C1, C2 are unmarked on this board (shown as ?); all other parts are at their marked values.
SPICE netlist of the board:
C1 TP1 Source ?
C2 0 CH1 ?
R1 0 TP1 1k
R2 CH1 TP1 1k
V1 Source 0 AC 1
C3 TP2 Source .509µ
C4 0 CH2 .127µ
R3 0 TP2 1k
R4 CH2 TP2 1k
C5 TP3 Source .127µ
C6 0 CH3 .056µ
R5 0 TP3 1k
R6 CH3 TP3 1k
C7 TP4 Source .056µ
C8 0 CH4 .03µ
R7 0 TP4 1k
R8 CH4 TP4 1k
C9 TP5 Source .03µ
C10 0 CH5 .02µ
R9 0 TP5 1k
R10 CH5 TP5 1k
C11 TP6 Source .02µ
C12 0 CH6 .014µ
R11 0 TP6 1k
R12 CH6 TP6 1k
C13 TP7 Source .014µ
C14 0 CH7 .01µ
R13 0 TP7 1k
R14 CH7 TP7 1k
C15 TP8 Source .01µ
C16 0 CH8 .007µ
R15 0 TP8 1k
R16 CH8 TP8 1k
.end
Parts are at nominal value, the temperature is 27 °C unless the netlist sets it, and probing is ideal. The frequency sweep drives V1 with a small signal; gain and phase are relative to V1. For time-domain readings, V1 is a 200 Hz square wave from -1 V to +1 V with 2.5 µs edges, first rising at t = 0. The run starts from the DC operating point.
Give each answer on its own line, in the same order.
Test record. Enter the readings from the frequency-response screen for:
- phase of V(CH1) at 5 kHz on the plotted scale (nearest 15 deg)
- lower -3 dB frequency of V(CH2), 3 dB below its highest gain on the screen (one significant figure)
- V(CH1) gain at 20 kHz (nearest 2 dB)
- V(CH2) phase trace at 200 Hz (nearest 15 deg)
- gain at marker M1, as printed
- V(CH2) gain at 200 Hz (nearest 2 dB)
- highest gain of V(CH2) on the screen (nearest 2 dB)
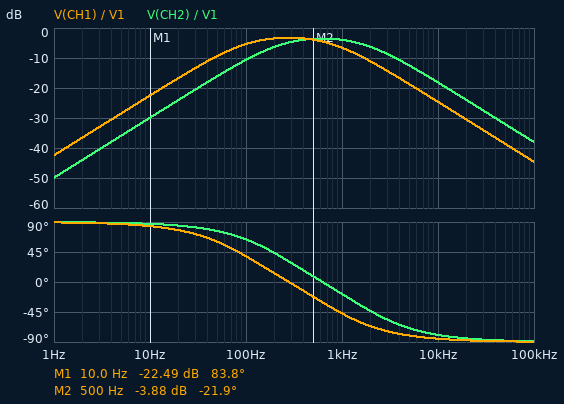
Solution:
-75 deg
200 Hz
-30 dB
45 deg
-22.49 dB
-6 dB
-4 dB
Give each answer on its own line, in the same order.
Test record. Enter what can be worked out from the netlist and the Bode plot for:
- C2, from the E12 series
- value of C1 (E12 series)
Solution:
270 nF
1.2 µF
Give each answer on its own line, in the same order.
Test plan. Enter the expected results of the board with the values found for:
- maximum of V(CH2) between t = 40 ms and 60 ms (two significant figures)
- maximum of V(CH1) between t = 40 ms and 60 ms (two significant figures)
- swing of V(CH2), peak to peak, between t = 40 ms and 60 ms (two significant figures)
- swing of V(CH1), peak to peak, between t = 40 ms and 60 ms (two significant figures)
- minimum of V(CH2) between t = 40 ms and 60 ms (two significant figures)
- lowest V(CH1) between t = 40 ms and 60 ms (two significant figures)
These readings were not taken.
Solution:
1.1 V
930 mV
2.1 V
1.9 V
-1.1 V
-930 mV
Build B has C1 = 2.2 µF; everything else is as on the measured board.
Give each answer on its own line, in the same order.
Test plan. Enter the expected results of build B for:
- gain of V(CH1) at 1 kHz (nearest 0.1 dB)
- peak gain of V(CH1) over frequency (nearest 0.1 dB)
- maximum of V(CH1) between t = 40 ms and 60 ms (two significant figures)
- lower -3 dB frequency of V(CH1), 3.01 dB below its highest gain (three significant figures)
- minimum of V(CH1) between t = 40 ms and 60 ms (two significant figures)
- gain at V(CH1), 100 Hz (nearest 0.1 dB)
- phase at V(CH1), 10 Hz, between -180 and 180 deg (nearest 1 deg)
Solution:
-6.2 dB
-1.9 dB
970 mV
54.1 Hz
-970 mV
-2.7 dB
80 deg
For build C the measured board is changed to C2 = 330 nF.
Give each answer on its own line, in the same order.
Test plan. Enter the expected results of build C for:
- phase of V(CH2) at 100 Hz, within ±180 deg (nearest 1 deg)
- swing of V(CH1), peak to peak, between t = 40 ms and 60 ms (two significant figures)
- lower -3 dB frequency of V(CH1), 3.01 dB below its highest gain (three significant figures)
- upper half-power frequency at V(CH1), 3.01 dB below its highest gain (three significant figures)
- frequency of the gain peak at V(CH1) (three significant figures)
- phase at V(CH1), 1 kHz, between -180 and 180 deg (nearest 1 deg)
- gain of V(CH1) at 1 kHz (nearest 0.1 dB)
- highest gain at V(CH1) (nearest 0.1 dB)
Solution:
64 deg
1.7 V
77.5 Hz
825 Hz
253 Hz
-51 deg
-7.9 dB
-3.8 dB
